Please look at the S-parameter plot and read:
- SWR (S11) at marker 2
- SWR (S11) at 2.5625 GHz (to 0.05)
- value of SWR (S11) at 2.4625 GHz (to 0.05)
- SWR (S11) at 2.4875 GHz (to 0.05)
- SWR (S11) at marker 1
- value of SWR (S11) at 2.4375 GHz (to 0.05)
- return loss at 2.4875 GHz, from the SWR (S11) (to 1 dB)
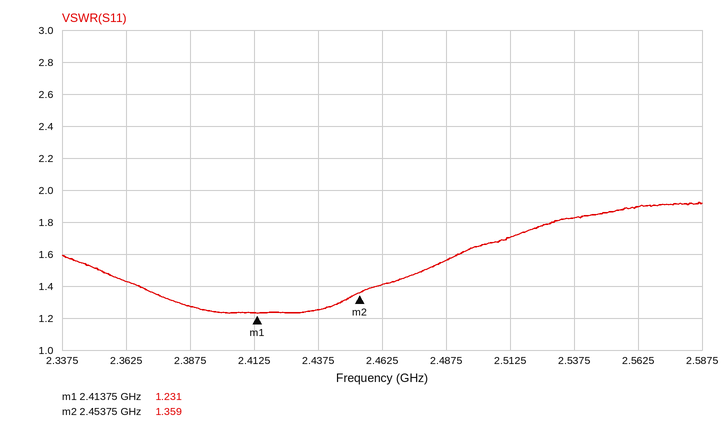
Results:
1.359
1.90
1.40
1.55
1.231
1.25
13 dB
